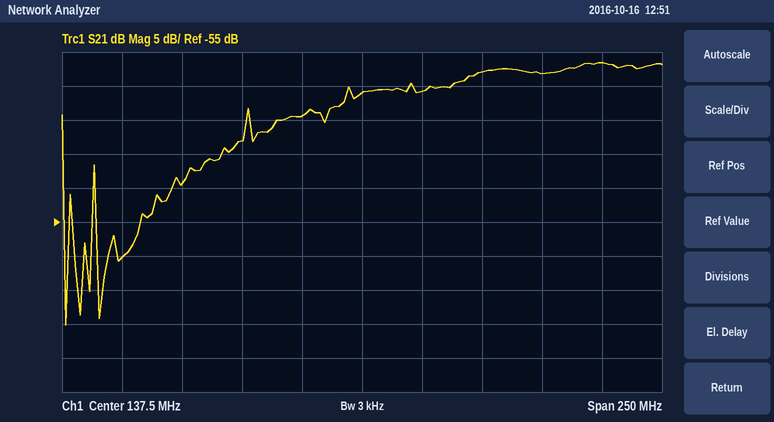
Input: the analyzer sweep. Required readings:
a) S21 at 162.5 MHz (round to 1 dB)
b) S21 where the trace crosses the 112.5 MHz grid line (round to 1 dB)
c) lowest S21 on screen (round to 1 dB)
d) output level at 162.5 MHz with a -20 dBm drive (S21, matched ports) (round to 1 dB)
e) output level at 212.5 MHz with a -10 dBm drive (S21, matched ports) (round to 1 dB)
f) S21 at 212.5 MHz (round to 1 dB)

-36 dB
-39 dB
-70 dB
-56 dBm
-43 dBm
-33 dB
